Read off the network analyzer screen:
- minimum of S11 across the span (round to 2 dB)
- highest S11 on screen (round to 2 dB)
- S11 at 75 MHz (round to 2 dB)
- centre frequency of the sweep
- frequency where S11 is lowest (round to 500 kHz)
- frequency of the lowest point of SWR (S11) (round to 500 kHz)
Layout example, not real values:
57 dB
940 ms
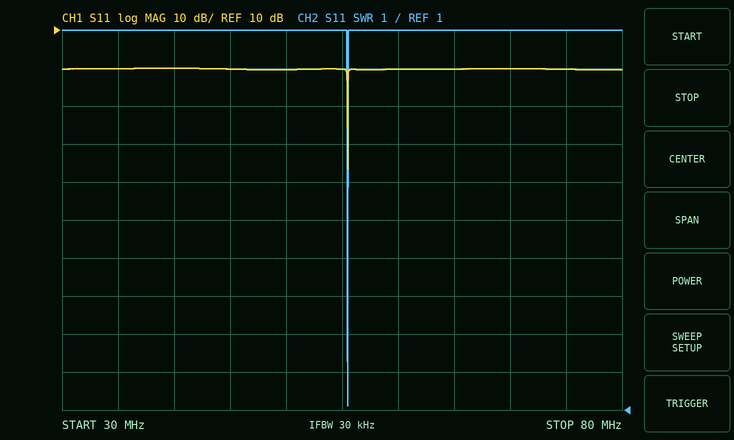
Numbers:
-26 dB
0 dB
0 dB
55 MHz
55.5 MHz
55.5 MHz
